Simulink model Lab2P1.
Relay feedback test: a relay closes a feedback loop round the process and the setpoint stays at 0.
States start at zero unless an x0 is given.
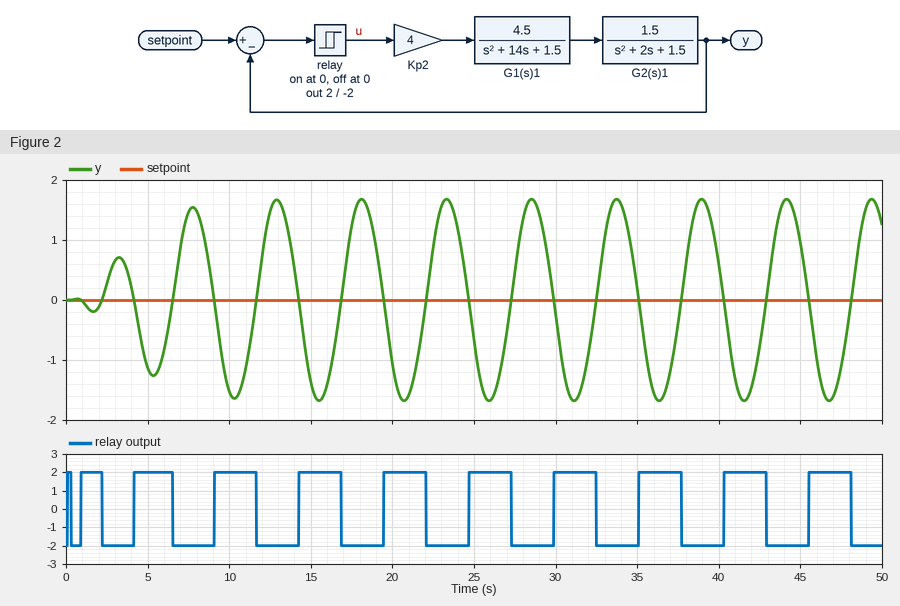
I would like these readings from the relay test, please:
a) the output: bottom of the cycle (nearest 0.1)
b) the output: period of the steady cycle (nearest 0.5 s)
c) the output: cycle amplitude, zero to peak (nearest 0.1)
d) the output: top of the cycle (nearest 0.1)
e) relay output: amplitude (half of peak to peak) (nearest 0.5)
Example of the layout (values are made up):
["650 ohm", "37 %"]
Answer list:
["-1.7", "5.0 s", "1.7", "1.7", "2.0"]
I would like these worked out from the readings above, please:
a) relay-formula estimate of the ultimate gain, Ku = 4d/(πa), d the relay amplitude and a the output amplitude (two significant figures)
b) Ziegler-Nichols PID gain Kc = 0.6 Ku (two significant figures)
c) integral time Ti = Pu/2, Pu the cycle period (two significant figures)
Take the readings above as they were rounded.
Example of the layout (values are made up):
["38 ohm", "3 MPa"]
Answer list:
["1.5", "0.90", "2.5 s"]
